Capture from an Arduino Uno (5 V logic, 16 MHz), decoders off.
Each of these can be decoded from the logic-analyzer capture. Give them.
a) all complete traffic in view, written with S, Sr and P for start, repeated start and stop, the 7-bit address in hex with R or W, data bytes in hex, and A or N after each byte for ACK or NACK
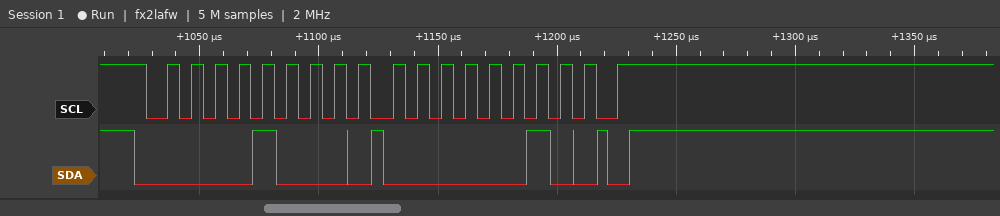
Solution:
S 04W A 02 A P
